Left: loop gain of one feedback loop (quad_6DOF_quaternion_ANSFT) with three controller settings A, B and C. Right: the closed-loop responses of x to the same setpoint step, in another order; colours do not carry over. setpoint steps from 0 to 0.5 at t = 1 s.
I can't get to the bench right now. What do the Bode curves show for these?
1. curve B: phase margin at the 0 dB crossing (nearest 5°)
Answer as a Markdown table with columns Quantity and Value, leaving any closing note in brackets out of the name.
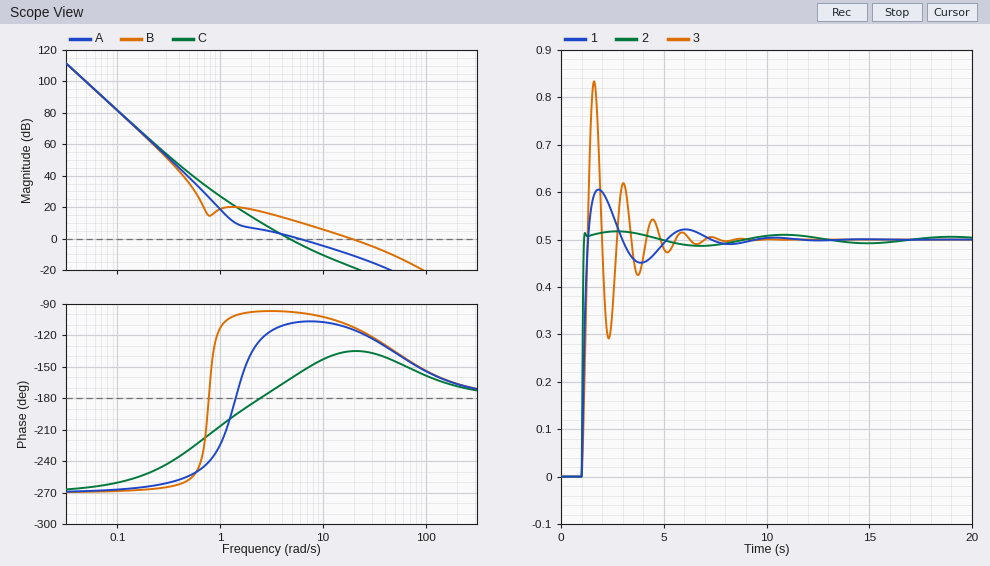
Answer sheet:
| Quantity | Value |
|---|---|
| curve B: phase margin at the 0 dB crossing | 70° |
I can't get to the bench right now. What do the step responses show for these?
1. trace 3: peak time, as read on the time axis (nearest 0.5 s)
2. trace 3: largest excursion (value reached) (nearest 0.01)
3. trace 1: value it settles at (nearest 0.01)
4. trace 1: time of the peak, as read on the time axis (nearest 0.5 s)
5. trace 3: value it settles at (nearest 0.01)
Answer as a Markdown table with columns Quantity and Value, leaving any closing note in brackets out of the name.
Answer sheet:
| Quantity | Value |
|---|---|
| trace 3: peak time, as read on the time axis | 1.5 s |
| trace 3: largest excursion (value reached) | 0.83 |
| trace 1: value it settles at | 0.50 |
| trace 1: time of the peak, as read on the time axis | 2.0 s |
| trace 3: value it settles at | 0.50 |
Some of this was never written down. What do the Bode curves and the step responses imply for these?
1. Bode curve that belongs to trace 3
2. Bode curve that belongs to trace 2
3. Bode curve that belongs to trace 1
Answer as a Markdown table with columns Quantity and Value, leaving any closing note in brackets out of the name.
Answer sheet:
| Quantity | Value |
|---|---|
| Bode curve that belongs to trace 3 | C |
| Bode curve that belongs to trace 2 | B |
| Bode curve that belongs to trace 1 | A |
